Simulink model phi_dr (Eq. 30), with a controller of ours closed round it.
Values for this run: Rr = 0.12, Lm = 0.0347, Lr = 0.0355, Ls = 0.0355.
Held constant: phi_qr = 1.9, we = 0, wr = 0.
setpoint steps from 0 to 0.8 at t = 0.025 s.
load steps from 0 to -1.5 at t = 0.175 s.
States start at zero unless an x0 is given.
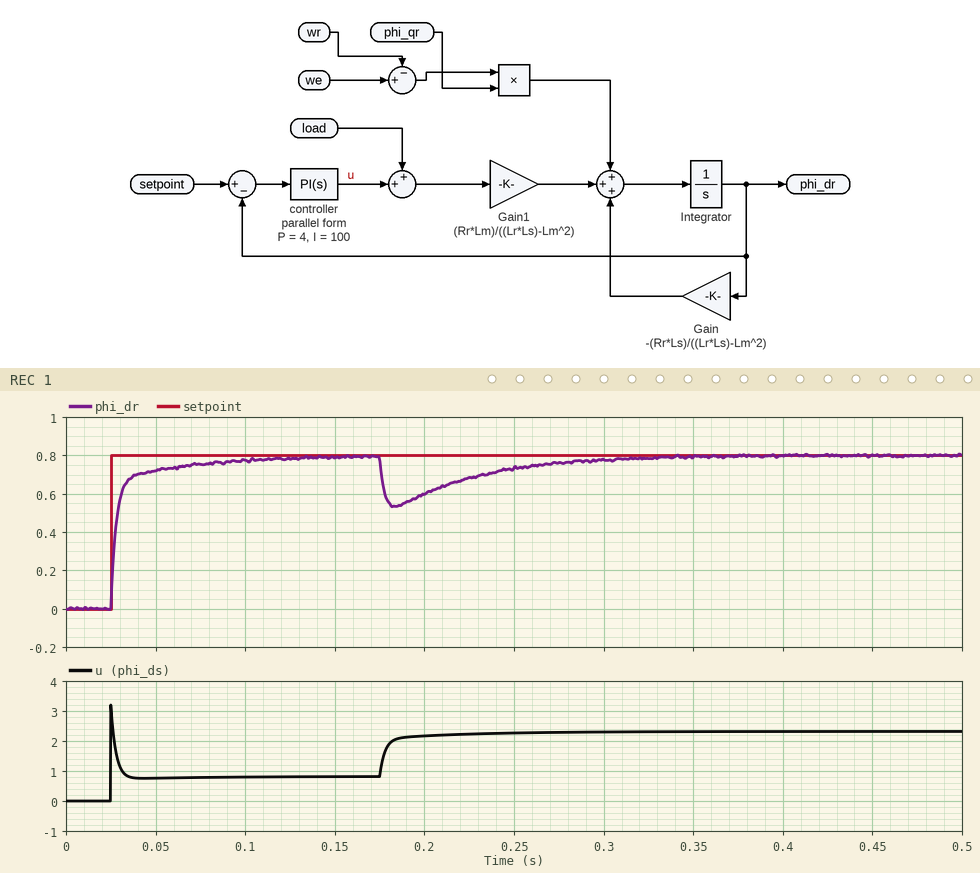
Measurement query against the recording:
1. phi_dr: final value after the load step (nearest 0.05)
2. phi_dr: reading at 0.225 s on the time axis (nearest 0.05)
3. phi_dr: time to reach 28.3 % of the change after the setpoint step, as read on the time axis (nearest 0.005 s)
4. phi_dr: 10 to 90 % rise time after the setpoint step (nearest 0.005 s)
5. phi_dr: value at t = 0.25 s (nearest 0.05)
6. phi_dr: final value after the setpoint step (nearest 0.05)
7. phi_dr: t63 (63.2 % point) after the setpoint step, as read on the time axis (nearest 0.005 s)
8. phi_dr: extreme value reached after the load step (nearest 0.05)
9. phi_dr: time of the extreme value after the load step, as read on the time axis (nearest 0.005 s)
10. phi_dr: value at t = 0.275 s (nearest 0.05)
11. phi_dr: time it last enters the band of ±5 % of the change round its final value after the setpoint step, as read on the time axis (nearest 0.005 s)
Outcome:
0.80
0.70
0.025 s
0.025 s
0.75
0.80
0.030 s
0.55
0.185 s
0.75
0.080 s
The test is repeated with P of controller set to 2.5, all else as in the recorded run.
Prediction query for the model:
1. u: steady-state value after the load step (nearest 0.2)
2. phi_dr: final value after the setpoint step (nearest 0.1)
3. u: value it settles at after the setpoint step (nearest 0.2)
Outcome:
2.4
0.8
0.8
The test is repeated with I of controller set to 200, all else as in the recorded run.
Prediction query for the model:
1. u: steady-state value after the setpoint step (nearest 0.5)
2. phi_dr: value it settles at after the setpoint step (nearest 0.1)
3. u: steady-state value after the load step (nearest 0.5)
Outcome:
1.0
0.8
2.5
